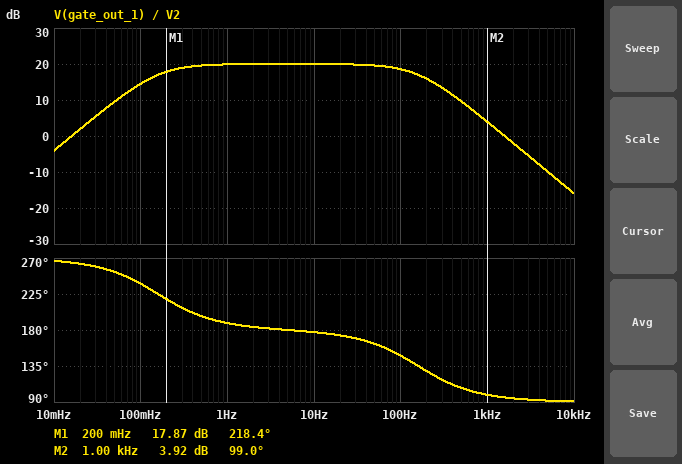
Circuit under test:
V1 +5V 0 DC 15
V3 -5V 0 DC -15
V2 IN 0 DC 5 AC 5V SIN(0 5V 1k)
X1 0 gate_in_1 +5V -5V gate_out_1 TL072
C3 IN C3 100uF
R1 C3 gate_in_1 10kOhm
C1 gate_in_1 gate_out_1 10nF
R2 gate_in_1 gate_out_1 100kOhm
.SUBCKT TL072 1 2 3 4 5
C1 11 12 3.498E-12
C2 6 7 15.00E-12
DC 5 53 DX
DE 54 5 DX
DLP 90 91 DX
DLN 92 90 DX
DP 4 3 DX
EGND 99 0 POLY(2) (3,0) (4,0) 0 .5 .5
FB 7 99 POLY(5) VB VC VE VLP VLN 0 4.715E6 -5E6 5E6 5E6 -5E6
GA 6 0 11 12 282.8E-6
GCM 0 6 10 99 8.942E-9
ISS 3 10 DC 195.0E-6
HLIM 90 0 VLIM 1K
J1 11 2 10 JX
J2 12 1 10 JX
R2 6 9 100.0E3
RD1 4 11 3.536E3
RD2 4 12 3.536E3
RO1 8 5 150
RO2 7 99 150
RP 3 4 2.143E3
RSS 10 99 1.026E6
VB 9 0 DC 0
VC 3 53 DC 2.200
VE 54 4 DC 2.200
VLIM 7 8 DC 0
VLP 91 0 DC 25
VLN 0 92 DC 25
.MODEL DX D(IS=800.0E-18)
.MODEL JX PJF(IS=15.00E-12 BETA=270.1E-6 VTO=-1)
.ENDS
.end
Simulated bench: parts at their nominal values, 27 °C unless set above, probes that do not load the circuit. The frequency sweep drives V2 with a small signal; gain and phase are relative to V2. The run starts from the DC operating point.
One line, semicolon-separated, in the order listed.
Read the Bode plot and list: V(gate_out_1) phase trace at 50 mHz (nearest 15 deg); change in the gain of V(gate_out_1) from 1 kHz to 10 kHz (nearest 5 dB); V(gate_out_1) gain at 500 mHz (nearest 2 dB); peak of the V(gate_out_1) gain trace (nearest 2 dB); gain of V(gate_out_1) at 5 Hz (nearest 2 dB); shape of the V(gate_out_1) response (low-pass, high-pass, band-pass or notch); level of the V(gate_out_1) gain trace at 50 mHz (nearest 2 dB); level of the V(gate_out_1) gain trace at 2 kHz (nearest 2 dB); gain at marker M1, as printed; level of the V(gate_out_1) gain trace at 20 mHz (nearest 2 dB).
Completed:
255 deg; -20 dB; 20 dB; 20 dB; 20 dB; band-pass; 10 dB; -2 dB; 17.87 dB; 2 dB
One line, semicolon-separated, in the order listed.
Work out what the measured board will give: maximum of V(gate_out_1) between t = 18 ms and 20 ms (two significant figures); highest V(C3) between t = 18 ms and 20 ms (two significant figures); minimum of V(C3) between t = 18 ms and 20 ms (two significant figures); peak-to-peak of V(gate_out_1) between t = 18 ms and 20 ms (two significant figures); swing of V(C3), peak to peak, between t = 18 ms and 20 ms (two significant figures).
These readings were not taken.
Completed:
7.9 V; 5.0 V; -5.0 V; 16 V; 10 V
